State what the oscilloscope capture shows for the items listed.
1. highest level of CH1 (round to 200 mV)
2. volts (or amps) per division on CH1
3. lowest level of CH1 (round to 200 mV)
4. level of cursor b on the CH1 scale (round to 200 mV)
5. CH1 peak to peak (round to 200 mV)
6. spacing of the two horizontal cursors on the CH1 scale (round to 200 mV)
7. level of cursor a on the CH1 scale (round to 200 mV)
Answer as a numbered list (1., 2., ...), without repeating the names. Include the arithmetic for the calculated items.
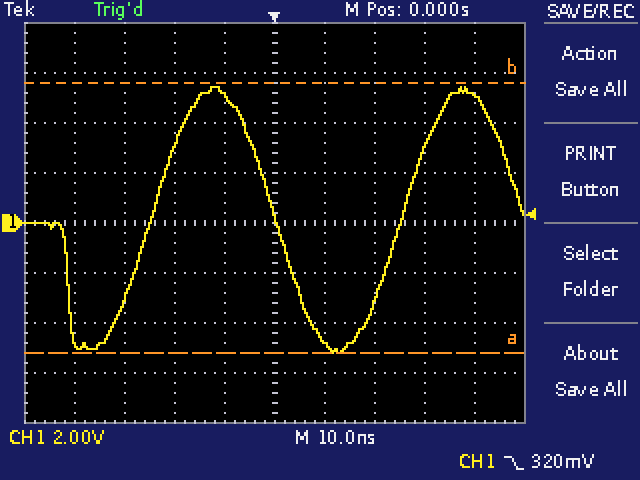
1. 5.4 V
2. 2 V
3. -5.2 V
4. 5.6 V
5. 5.4 V − (-5.2 V) = 10.6 V
6. 10.8 V
7. -5.2 V
